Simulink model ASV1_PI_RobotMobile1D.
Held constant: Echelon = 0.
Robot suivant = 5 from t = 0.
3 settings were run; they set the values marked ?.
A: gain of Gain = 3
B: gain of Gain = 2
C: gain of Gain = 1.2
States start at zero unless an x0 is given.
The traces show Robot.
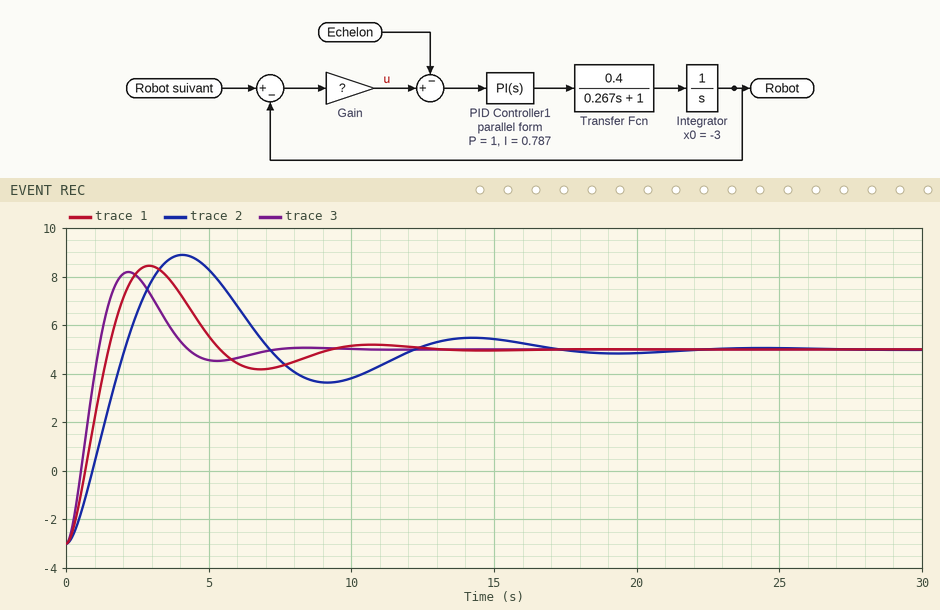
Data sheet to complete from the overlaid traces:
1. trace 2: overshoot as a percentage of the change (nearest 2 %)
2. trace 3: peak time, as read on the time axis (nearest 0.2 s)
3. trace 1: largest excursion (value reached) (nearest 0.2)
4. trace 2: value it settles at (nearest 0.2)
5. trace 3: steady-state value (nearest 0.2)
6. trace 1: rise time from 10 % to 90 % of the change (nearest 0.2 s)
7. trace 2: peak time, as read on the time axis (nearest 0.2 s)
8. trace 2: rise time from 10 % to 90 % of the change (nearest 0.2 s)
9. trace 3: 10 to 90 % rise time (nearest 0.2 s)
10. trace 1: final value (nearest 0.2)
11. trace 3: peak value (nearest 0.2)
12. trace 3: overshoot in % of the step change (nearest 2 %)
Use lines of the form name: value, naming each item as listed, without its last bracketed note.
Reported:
trace 2: overshoot as a percentage of the change: 48 %
trace 3: peak time, as read on the time axis: 2.2 s
trace 1: largest excursion (value reached): 8.4
trace 2: value it settles at: 5.0
trace 3: steady-state value: 5.0
trace 1: rise time from 10 % to 90 % of the change: 1.0 s
trace 2: peak time, as read on the time axis: 4.0 s
trace 2: rise time from 10 % to 90 % of the change: 1.4 s
trace 3: 10 to 90 % rise time: 0.8 s
trace 1: final value: 5.0
trace 3: peak value: 8.2
trace 3: overshoot in % of the step change: 40 %
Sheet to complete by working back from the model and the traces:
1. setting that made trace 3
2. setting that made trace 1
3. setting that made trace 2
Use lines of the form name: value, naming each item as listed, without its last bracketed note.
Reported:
setting that made trace 3: A
setting that made trace 1: B
setting that made trace 2: C
